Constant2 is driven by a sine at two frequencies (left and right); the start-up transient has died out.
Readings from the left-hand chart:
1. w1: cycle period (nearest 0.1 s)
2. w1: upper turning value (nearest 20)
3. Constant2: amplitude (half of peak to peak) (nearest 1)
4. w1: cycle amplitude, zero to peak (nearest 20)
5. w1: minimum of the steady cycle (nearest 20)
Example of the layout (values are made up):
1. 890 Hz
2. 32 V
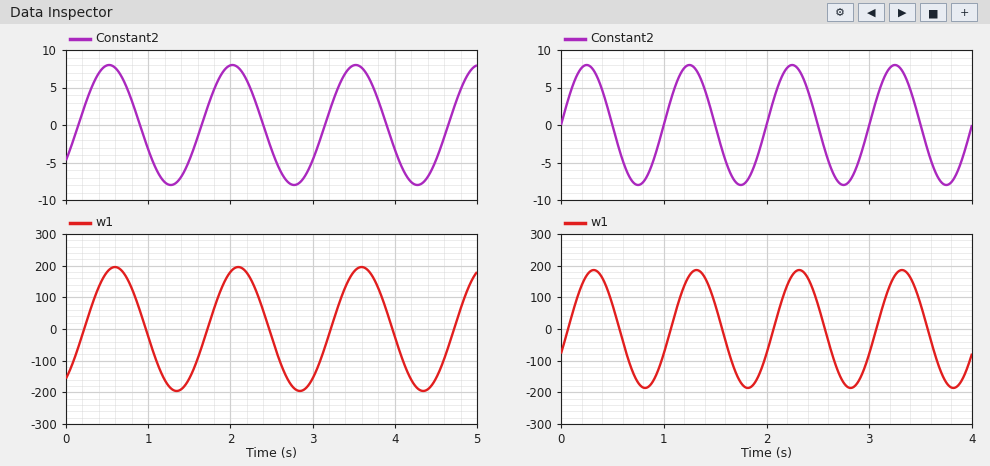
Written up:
1. 1.5 s
2. 200
3. 8
4. 200
5. -200
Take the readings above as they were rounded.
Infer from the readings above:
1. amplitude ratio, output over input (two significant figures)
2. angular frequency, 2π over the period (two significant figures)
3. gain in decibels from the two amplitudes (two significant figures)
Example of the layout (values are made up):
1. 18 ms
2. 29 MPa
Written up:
1. 25
2. 4.2 rad/s
3. 28 dB
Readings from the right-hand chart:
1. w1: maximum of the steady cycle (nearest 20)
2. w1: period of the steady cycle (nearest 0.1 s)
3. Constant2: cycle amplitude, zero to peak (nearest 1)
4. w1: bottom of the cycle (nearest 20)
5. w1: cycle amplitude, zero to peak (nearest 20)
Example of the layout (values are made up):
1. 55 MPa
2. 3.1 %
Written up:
1. 180
2. 1.0 s
3. 8
4. -180
5. 180
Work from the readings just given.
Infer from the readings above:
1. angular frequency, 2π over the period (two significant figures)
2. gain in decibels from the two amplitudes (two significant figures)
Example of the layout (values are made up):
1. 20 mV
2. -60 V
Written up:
1. 6.3 rad/s
2. 27 dB
